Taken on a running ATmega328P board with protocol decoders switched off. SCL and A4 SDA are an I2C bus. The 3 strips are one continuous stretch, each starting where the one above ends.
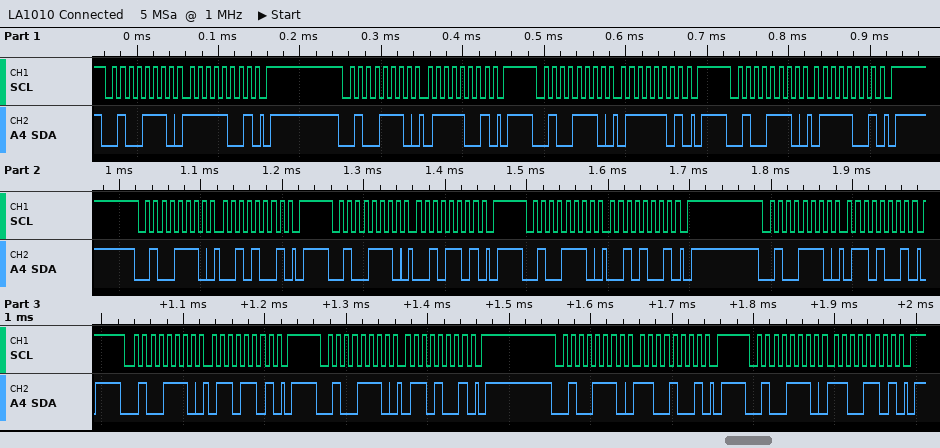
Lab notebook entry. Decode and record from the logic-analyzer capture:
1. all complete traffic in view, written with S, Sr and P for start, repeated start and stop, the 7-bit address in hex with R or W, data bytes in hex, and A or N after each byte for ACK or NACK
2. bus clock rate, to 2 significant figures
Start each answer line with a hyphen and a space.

- S 27W A F9 A P S 27W A 79 A P S 27W A 7D A P S 27W A 79 A P S 27W A 29 A P S 27W A 2D A P S 27W A 29 A P S 27W A 69 A P S 27W A 6D A P S 27W A 69 A P S 27W A C9 A P S 27W A CD A P
- 100 kHz
